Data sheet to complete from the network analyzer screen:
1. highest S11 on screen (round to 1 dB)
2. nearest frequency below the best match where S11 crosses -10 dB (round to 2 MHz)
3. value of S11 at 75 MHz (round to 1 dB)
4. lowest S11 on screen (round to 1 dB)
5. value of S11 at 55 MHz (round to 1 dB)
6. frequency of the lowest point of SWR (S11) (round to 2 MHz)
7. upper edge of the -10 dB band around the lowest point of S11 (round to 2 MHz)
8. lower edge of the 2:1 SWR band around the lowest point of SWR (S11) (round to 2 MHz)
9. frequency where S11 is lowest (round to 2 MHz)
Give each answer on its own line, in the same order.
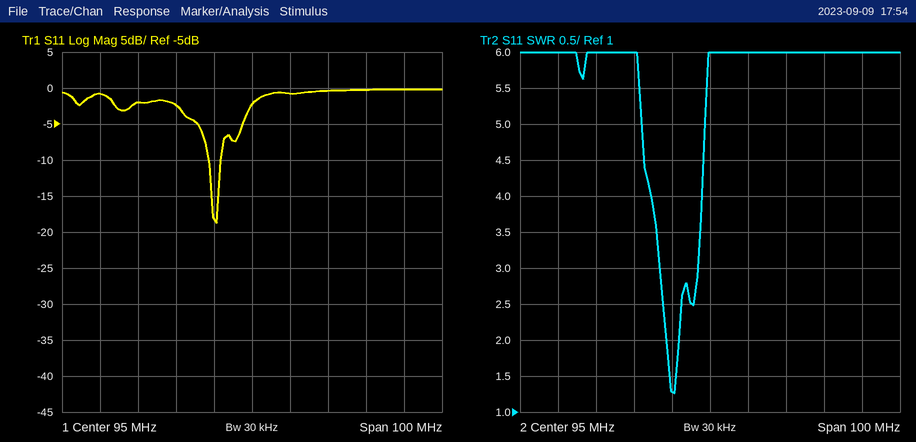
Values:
0 dB
84 MHz
-2 dB
-19 dB
-1 dB
86 MHz
86 MHz
84 MHz
86 MHz
